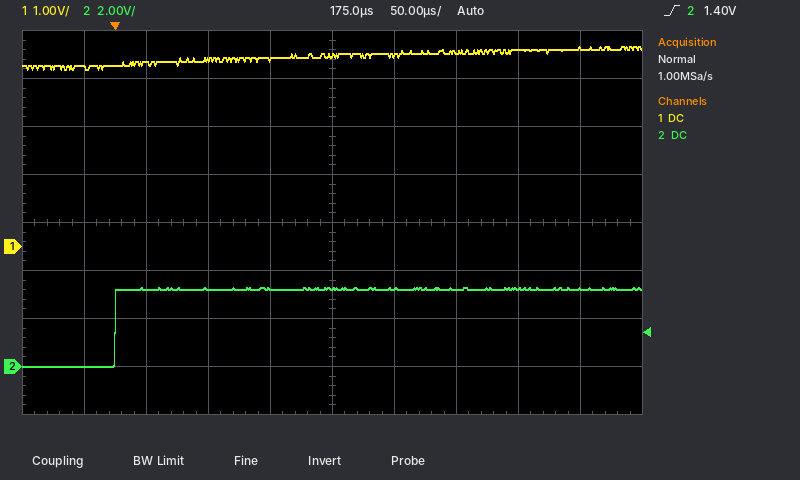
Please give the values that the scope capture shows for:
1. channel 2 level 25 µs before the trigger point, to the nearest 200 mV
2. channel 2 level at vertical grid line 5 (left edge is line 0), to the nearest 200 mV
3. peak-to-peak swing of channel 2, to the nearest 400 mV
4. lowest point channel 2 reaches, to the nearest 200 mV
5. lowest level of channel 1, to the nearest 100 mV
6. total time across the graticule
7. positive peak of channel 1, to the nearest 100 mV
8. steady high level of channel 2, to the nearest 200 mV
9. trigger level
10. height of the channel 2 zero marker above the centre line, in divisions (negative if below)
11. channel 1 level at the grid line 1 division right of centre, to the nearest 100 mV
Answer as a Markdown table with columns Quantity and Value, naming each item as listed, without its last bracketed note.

| Quantity | Value |
|---|---|
| channel 2 level 25 µs before the trigger point, to the nearest 200 mV | 0.0 V |
| channel 2 level at vertical grid line 5 (left edge is line 0), to the nearest 200 mV | 3.2 V |
| peak-to-peak swing of channel 2, to the nearest 400 mV | 3.2 V |
| lowest point channel 2 reaches, to the nearest 200 mV | 0.0 V |
| lowest level of channel 1, to the nearest 100 mV | 3.7 V |
| total time across the graticule | 500 µs |
| positive peak of channel 1, to the nearest 100 mV | 4.2 V |
| steady high level of channel 2, to the nearest 200 mV | 3.2 V |
| trigger level | 1.40 V |
| height of the channel 2 zero marker above the centre line, in divisions | -3.0 div |
| channel 1 level at the grid line 1 division right of centre, to the nearest 100 mV | 4.0 V |
